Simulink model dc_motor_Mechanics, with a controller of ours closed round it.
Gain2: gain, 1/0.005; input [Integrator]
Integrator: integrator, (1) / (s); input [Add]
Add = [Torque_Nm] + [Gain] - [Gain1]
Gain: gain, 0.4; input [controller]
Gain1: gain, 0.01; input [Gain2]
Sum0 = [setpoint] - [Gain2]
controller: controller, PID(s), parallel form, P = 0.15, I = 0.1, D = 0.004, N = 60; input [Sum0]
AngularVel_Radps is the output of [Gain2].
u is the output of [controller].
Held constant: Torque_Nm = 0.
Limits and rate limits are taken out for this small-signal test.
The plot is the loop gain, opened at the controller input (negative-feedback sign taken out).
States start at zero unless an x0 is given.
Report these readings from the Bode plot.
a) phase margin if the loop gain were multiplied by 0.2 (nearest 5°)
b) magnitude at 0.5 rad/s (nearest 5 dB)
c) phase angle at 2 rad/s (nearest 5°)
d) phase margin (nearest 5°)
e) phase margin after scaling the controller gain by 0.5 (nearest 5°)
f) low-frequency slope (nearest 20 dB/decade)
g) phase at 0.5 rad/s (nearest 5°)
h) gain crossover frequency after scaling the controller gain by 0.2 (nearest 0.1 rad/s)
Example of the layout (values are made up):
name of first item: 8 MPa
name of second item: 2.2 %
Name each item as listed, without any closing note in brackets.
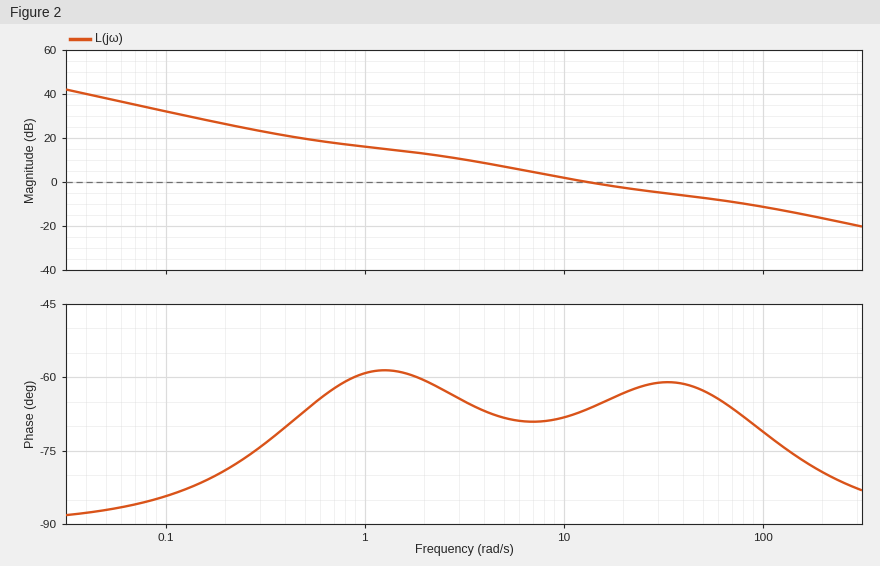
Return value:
phase margin if the loop gain were multiplied by 0.2: 120°
magnitude at 0.5 rad/s: 20 dB
phase angle at 2 rad/s: -60°
phase margin: 115°
phase margin after scaling the controller gain by 0.5: 110°
low-frequency slope: -20 dB/decade
phase at 0.5 rad/s: -65°
gain crossover frequency after scaling the controller gain by 0.2: 1.6 rad/s
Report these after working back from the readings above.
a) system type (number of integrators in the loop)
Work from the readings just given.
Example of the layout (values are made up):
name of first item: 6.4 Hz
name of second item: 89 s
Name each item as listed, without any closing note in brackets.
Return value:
system type: 1
